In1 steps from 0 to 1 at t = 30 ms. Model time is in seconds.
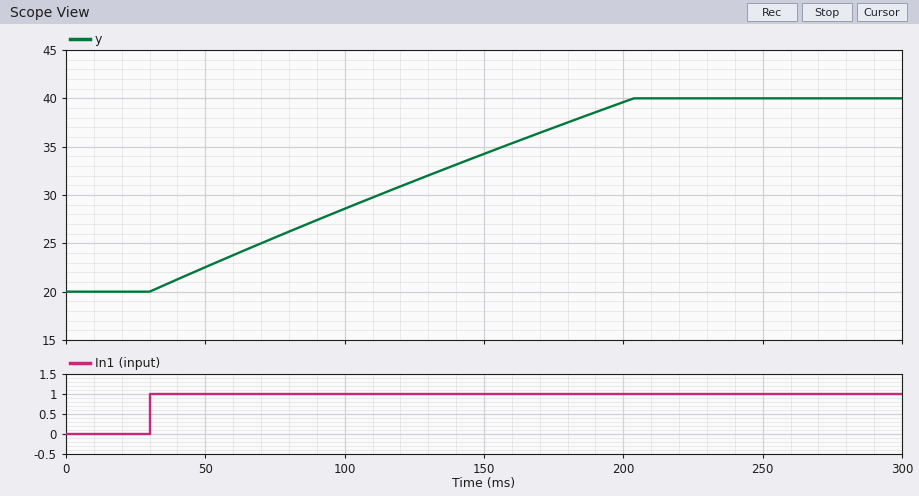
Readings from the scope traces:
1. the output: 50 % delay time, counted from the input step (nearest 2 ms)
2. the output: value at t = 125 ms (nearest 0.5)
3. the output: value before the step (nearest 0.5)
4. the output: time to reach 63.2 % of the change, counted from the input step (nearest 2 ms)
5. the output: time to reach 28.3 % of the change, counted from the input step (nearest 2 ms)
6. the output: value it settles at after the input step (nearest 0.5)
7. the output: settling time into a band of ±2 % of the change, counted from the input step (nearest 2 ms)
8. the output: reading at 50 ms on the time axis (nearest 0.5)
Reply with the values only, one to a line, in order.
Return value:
82 ms
31.5
20.0
106 ms
46 ms
40.0
170 ms
22.5
